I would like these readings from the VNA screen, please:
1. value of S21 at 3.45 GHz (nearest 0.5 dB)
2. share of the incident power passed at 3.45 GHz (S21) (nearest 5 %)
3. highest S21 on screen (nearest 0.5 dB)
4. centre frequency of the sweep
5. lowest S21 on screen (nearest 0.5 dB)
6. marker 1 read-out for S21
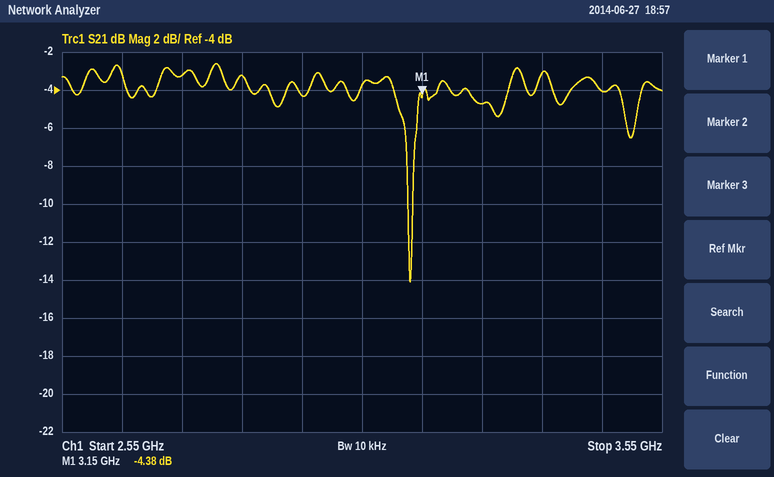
-4.0 dB
40 %
-2.5 dB
3.05 GHz
-14.0 dB
-4.38 dB
